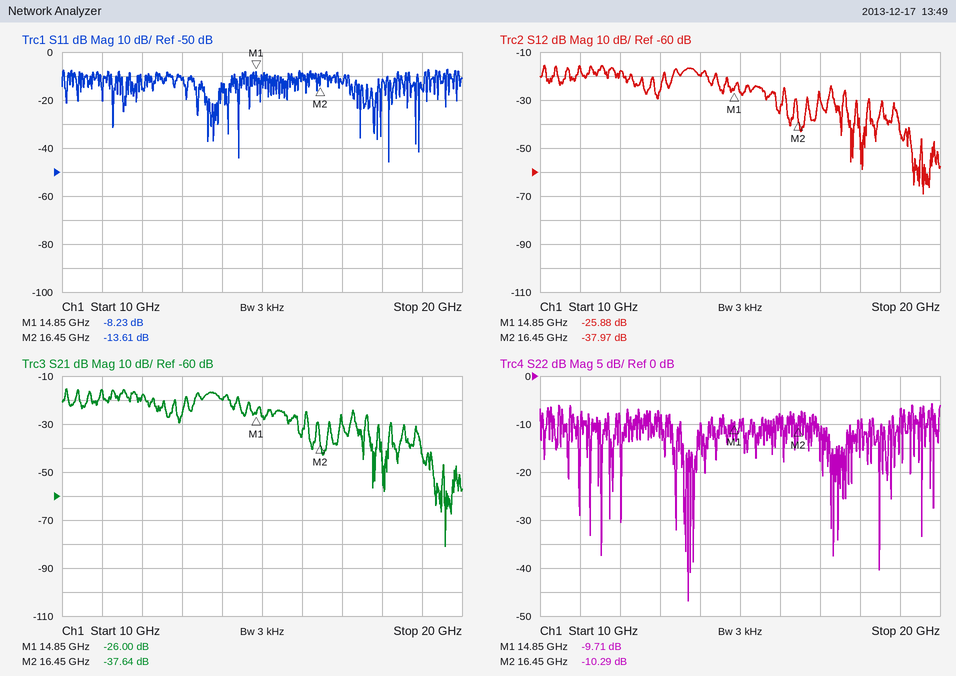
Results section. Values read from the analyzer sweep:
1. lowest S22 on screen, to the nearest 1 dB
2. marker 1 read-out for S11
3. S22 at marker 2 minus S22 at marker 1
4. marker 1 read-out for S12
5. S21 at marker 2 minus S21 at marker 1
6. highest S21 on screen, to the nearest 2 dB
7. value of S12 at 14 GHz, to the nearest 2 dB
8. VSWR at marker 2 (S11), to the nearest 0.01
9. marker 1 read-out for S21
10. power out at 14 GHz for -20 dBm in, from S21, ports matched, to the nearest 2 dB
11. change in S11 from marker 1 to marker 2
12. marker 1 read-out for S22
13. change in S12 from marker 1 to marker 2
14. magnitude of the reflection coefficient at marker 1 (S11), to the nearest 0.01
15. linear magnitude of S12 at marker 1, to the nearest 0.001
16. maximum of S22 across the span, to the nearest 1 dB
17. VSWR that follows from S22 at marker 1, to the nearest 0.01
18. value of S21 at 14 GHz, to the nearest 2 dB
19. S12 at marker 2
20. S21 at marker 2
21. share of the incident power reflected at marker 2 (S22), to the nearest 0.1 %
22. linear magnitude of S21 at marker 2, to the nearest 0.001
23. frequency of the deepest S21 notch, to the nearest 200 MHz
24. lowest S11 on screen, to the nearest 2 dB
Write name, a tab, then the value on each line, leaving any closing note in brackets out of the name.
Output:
lowest S22 on screen, to the nearest 1 dB	-47 dB
marker 1 read-out for S11	-8.23 dB
S22 at marker 2 minus S22 at marker 1	-0.58 dB
marker 1 read-out for S12	-25.88 dB
S21 at marker 2 minus S21 at marker 1	-11.64 dB
highest S21 on screen, to the nearest 2 dB	-16 dB
value of S12 at 14 GHz, to the nearest 2 dB	-20 dB
VSWR at marker 2 (S11), to the nearest 0.01	1.53
marker 1 read-out for S21	-26.00 dB
power out at 14 GHz for -20 dBm in, from S21, ports matched, to the nearest 2 dB	-40 dBm
change in S11 from marker 1 to marker 2	-5.38 dB
marker 1 read-out for S22	-9.71 dB
change in S12 from marker 1 to marker 2	-12.09 dB
magnitude of the reflection coefficient at marker 1 (S11), to the nearest 0.01	0.39
linear magnitude of S12 at marker 1, to the nearest 0.001	0.051
maximum of S22 across the span, to the nearest 1 dB	-6 dB
VSWR that follows from S22 at marker 1, to the nearest 0.01	1.97
value of S21 at 14 GHz, to the nearest 2 dB	-20 dB
S12 at marker 2	-37.97 dB
S21 at marker 2	-37.64 dB
share of the incident power reflected at marker 2 (S22), to the nearest 0.1 %	9.4 %
linear magnitude of S21 at marker 2, to the nearest 0.001	0.013
frequency of the deepest S21 notch, to the nearest 200 MHz	19.6 GHz
lowest S11 on screen, to the nearest 2 dB	-46 dB
